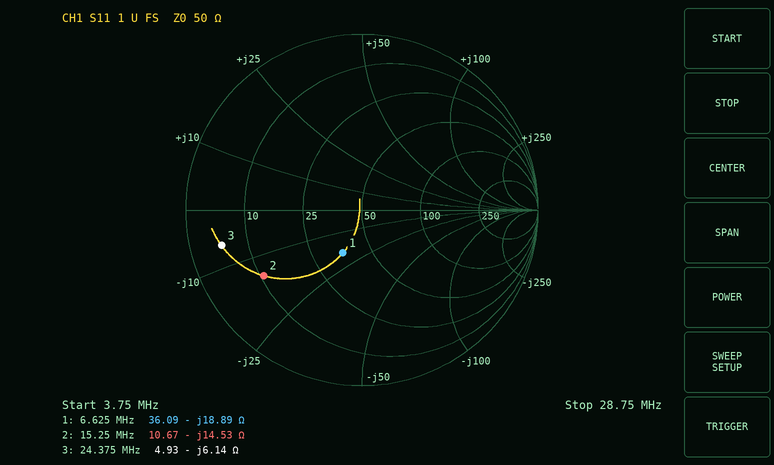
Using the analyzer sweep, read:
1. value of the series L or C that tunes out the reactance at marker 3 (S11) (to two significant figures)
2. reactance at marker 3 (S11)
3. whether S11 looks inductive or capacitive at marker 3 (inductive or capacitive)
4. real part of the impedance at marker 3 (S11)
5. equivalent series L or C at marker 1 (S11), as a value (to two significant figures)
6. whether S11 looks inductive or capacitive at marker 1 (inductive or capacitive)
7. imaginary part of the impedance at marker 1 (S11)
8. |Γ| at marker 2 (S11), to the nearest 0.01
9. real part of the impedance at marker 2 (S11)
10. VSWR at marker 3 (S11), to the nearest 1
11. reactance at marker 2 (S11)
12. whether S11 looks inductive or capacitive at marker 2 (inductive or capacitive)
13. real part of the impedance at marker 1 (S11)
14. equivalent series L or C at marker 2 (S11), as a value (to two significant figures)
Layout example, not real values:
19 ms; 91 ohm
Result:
40 nH; -6.14 Ω; capacitive; 4.93 Ω; 1.3 nF; capacitive; -18.89 Ω; 0.67; 10.67 Ω; 10; -14.53 Ω; capacitive; 36.09 Ω; 720 pF
